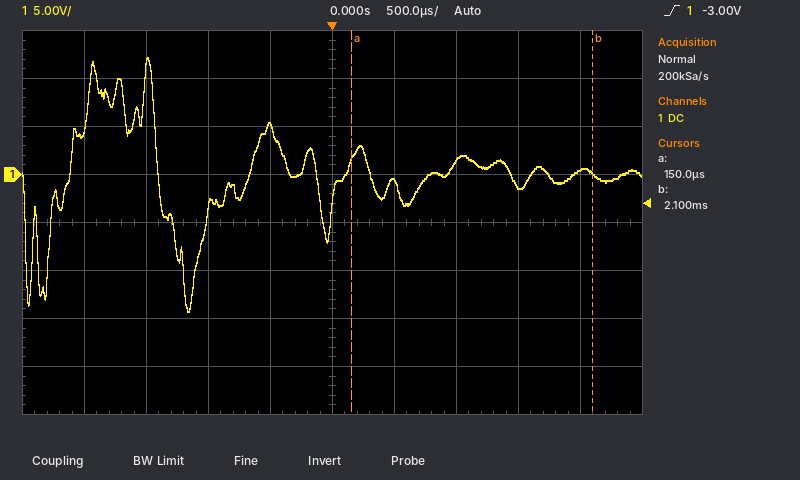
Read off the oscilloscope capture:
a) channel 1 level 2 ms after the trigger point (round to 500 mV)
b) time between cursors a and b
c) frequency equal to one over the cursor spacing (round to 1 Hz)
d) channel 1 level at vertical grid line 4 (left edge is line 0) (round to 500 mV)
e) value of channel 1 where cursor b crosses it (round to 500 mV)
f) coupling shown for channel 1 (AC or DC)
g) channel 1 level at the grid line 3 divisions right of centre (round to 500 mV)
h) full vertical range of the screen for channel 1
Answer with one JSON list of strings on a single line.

["500 mV", "1.95 ms", "513 Hz", "5.0 V", "0.0 V", "DC", "-1.0 V", "40 V"]
